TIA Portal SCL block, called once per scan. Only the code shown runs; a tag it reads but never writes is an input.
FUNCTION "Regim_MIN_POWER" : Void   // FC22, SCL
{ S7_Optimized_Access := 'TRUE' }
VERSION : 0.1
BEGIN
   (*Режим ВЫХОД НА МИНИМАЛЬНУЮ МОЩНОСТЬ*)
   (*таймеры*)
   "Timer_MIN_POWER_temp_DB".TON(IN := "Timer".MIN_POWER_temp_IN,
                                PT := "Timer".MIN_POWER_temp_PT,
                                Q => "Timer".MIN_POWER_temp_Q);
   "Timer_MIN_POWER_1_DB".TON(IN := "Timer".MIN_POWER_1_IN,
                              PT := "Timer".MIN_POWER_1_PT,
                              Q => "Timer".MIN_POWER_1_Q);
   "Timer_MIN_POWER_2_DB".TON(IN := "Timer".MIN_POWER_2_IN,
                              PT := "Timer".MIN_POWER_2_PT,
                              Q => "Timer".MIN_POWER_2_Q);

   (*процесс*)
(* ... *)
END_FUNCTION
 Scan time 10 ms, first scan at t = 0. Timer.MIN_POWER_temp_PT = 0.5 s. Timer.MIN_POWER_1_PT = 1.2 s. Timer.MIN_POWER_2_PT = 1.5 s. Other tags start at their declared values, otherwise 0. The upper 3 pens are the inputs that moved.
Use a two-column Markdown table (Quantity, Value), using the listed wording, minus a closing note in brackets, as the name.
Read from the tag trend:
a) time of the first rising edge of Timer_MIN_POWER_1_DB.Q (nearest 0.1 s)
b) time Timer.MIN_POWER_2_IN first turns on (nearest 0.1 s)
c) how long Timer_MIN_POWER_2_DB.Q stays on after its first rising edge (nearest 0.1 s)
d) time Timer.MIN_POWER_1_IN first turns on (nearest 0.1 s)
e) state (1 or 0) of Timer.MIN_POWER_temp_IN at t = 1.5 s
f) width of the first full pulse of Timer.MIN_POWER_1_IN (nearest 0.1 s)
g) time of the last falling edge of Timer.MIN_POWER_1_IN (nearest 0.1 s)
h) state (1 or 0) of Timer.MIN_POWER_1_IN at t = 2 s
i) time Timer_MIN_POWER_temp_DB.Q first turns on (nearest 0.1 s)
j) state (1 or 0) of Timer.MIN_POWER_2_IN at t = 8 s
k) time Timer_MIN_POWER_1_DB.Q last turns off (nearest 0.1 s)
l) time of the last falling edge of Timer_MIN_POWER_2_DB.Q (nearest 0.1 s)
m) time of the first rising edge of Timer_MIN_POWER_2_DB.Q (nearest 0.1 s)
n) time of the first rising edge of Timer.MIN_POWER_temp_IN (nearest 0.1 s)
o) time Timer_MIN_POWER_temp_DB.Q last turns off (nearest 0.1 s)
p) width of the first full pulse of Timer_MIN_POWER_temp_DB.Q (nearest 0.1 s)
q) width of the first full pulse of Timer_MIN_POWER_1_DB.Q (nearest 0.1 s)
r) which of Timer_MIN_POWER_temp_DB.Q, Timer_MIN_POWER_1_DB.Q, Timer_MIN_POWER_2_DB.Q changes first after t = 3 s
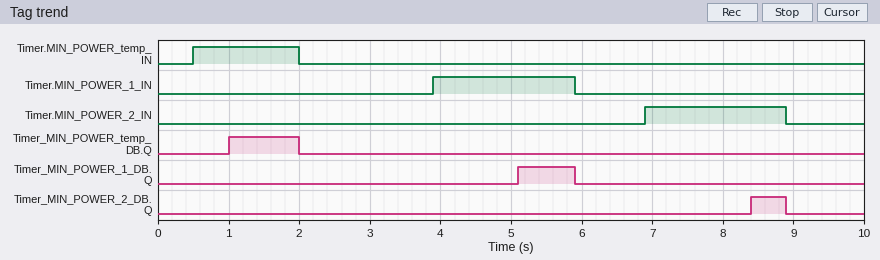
| Quantity | Value |
|---|---|
| time of the first rising edge of Timer_MIN_POWER_1_DB.Q | 5.1 s |
| time Timer.MIN_POWER_2_IN first turns on | 6.9 s |
| how long Timer_MIN_POWER_2_DB.Q stays on after its first rising edge | 0.5 s |
| time Timer.MIN_POWER_1_IN first turns on | 3.9 s |
| state (1 or 0) of Timer.MIN_POWER_temp_IN at t = 1.5 s | 1 |
| width of the first full pulse of Timer.MIN_POWER_1_IN | 2.0 s |
| time of the last falling edge of Timer.MIN_POWER_1_IN | 5.9 s |
| state (1 or 0) of Timer.MIN_POWER_1_IN at t = 2 s | 0 |
| time Timer_MIN_POWER_temp_DB.Q first turns on | 1.0 s |
| state (1 or 0) of Timer.MIN_POWER_2_IN at t = 8 s | 1 |
| time Timer_MIN_POWER_1_DB.Q last turns off | 5.9 s |
| time of the last falling edge of Timer_MIN_POWER_2_DB.Q | 8.9 s |
| time of the first rising edge of Timer_MIN_POWER_2_DB.Q | 8.4 s |
| time of the first rising edge of Timer.MIN_POWER_temp_IN | 0.5 s |
| time Timer_MIN_POWER_temp_DB.Q last turns off | 2.0 s |
| width of the first full pulse of Timer_MIN_POWER_temp_DB.Q | 1.0 s |
| width of the first full pulse of Timer_MIN_POWER_1_DB.Q | 0.8 s |
| which of Timer_MIN_POWER_temp_DB.Q, Timer_MIN_POWER_1_DB.Q, Timer_MIN_POWER_2_DB.Q changes first after t = 3 s | Timer_MIN_POWER_1_DB.Q |
